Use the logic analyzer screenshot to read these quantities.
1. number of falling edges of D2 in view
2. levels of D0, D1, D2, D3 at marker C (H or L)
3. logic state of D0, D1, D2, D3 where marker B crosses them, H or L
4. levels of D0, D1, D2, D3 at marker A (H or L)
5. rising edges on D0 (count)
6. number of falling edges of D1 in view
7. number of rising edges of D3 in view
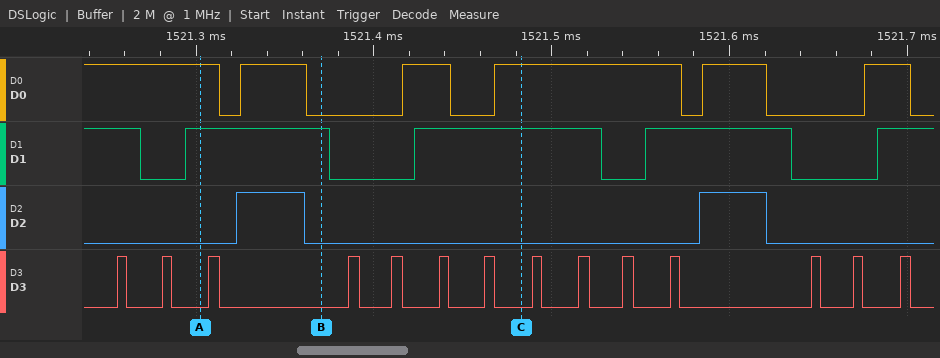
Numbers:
2
D0=H, D1=H, D2=L, D3=L
D0=L, D1=H, D2=L, D3=L
D0=H, D1=H, D2=L, D3=L
5
4
14
